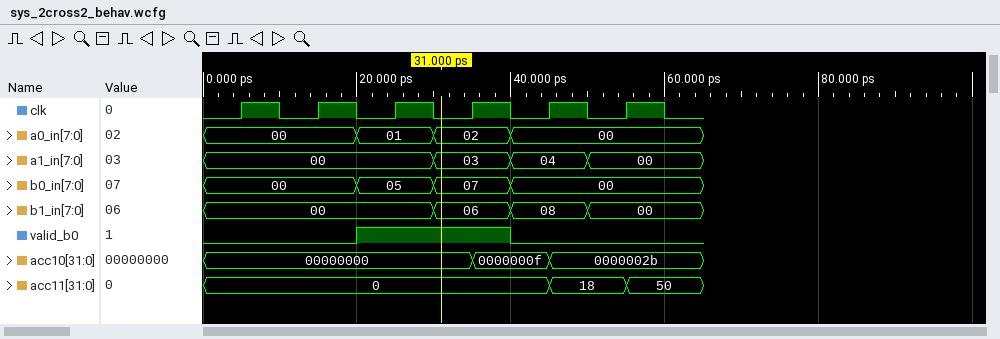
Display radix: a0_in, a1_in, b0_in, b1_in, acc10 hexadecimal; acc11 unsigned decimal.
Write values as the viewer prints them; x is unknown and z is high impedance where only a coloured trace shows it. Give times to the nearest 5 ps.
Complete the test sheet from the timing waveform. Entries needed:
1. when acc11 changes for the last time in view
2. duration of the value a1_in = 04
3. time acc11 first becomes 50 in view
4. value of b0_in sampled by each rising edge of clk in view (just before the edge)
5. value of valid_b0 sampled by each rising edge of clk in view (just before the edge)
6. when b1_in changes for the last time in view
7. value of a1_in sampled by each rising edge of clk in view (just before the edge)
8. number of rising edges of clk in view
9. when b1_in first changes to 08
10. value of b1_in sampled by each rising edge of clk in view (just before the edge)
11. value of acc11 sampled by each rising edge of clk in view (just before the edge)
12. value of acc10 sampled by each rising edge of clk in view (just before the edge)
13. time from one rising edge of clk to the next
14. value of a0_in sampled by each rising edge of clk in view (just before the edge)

55 ps
10 ps
55 ps
00, 00, 05, 07, 00, 00
0 0 1 1 0 0
50 ps
00, 00, 00, 03, 04, 00
6
40 ps
00, 00, 00, 06, 08, 00
0, 0, 0, 0, 0, 18
00000000, 00000000, 00000000, 00000000, 0000000f, 0000002b
10 ps
00, 00, 01, 02, 00, 00
